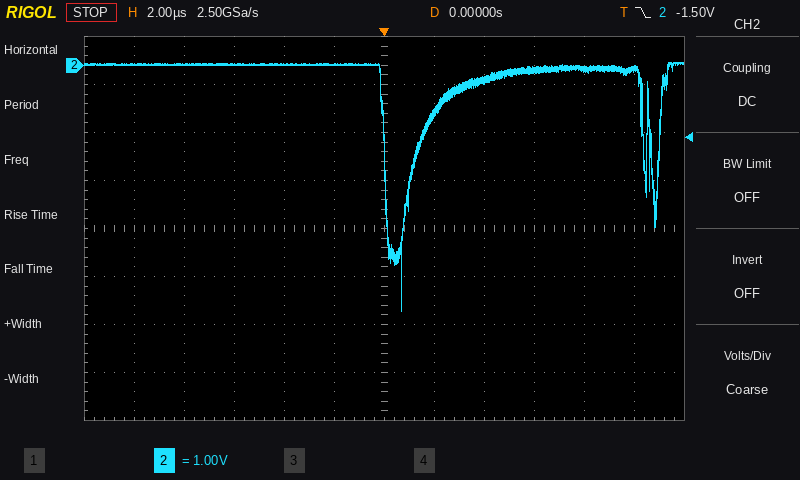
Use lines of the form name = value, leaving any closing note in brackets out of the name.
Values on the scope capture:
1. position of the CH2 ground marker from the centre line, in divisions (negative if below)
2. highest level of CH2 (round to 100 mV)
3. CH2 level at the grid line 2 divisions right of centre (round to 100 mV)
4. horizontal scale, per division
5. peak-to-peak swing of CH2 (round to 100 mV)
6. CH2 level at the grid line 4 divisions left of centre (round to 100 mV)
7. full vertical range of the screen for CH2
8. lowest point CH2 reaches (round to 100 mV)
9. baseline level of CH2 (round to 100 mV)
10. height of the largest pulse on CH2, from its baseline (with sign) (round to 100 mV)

position of the CH2 ground marker from the centre line, in divisions = +3.4 div
highest level of CH2 = 100 mV
CH2 level at the grid line 2 divisions right of centre = -300 mV
horizontal scale, per division = 2 µs
peak-to-peak swing of CH2 = 5.2 V
CH2 level at the grid line 4 divisions left of centre = 0.0 V
full vertical range of the screen for CH2 = 8 V
lowest point CH2 reaches = -5.1 V
baseline level of CH2 = 0.0 V
height of the largest pulse on CH2, from its baseline (with sign) = -5.1 V
